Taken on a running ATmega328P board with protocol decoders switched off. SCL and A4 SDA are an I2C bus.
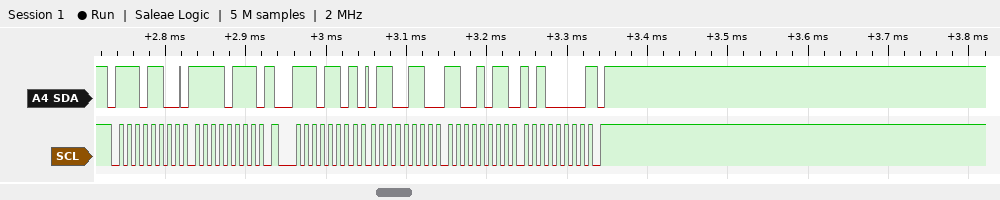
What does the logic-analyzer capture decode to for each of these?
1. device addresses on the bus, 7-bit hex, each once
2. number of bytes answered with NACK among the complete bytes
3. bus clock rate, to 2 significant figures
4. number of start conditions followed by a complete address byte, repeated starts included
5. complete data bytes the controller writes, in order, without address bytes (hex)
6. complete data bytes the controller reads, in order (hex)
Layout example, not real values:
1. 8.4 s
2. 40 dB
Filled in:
1. 0x76
2. 1
3. 100 kHz
4. 2
5. F7
6. 66 CB A0
